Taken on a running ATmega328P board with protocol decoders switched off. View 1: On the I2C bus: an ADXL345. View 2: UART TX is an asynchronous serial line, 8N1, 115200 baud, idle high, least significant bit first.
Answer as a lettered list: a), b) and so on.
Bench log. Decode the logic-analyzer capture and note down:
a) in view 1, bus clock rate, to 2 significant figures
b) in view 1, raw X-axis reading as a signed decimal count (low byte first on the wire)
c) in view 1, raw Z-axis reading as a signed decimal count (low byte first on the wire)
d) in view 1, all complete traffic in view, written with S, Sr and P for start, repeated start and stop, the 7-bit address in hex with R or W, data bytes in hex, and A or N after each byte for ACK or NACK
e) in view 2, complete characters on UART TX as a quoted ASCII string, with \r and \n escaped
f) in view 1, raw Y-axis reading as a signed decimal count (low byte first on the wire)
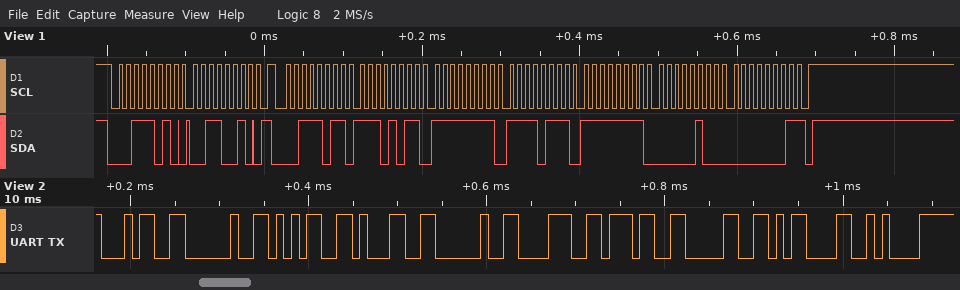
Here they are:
a) 100 kHz
b) -21
c) 260
d) S 1DW A 32 A Sr 1DR A EB A FF A F7 A FF A 04 A 01 N P
e) "4 51 870\r\n"
f) -9
